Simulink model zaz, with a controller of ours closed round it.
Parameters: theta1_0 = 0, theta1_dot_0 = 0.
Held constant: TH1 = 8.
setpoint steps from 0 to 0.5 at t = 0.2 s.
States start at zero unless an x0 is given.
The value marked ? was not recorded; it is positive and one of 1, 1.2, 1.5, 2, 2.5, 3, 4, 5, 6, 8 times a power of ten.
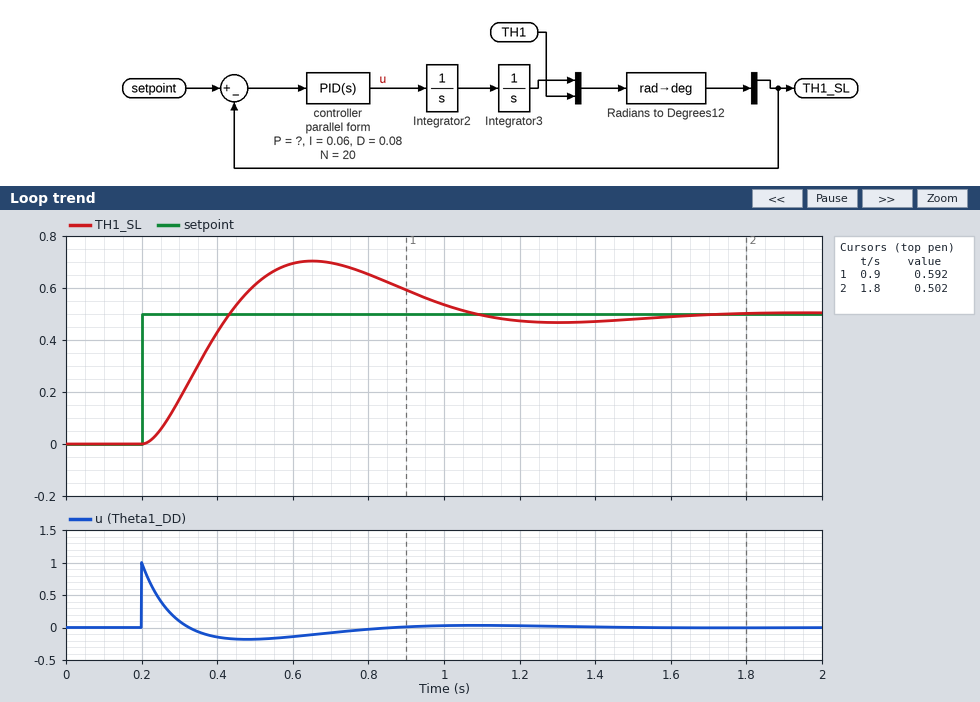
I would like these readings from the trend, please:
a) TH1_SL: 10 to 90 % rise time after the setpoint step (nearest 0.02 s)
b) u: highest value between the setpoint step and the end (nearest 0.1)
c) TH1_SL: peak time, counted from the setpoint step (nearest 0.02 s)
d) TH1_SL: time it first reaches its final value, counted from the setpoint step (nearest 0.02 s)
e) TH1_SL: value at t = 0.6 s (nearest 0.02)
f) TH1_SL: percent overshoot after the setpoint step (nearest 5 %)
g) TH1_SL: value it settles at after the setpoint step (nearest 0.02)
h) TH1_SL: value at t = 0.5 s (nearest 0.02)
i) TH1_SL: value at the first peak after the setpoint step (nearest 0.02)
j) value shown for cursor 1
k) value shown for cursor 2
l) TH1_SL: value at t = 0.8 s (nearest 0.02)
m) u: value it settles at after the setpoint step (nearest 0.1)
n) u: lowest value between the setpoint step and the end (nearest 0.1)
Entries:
0.16 s
1.0
0.46 s
0.24 s
0.70
40 %
0.50
0.62
0.70
0.592
0.502
0.66
0.0
-0.2
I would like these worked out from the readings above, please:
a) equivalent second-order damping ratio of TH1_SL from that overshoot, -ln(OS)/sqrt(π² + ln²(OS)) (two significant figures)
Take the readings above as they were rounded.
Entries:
0.28
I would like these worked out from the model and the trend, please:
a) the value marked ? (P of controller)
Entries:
0.4
